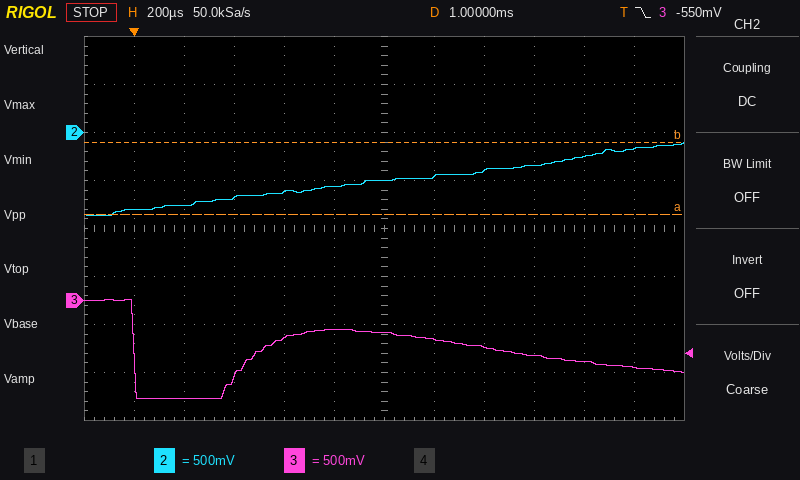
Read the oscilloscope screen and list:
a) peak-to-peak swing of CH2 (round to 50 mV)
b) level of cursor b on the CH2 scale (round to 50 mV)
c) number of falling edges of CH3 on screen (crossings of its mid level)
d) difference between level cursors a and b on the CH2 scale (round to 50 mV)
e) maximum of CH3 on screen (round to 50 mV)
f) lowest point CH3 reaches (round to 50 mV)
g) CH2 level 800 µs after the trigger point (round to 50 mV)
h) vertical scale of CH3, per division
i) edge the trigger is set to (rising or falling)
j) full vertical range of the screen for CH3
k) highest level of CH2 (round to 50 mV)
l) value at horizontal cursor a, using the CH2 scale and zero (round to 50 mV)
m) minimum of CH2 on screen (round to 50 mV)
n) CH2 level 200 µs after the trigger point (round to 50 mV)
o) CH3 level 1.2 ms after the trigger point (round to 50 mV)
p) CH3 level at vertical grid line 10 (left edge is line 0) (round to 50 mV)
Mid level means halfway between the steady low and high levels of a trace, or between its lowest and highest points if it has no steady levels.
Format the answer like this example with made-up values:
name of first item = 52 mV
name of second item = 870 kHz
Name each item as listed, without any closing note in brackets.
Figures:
peak-to-peak swing of CH2 = 750 mV
level of cursor b on the CH2 scale = -100 mV
number of falling edges of CH3 on screen = 2
difference between level cursors a and b on the CH2 scale = 750 mV
maximum of CH3 on screen = 0 mV
lowest point CH3 reaches = -1.00 V
CH2 level 800 µs after the trigger point = -550 mV
vertical scale of CH3, per division = 500 mV
edge the trigger is set to = falling
full vertical range of the screen for CH3 = 4 V
highest level of CH2 = -100 mV
value at horizontal cursor a, using the CH2 scale and zero = -850 mV
minimum of CH2 on screen = -850 mV
CH2 level 200 µs after the trigger point = -750 mV
CH3 level 1.2 ms after the trigger point = -400 mV
CH3 level at vertical grid line 10 (left edge is line 0) = -650 mV
